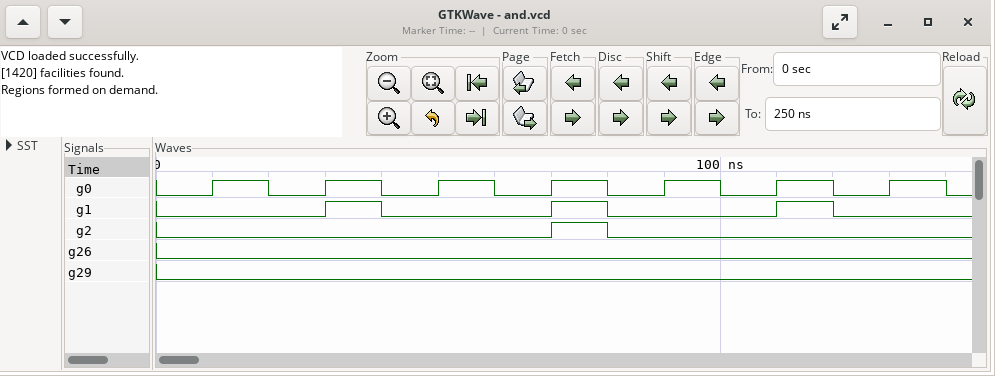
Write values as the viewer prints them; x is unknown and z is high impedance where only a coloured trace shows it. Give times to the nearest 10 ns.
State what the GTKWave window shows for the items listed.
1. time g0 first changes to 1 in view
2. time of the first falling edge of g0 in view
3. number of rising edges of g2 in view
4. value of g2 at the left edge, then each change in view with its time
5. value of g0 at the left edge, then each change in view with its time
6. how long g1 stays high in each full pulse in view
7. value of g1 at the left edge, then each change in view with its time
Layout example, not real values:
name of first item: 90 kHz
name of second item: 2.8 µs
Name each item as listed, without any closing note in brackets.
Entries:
time g0 first changes to 1 in view: 10 ns
time of the first falling edge of g0 in view: 20 ns
number of rising edges of g2 in view: 1
value of g2 at the left edge, then each change in view with its time: 0, 1 at 70 ns, 0 at 80 ns
value of g0 at the left edge, then each change in view with its time: 0, 1 at 10 ns, 0 at 20 ns, 1 at 30 ns, 0 at 40 ns, 1 at 50 ns, 0 at 60 ns, 1 at 70 ns, 0 at 80 ns, 1 at 90 ns, 0 at 100 ns, 1 at 110 ns, 0 at 120 ns, 1 at 130 ns, 0 at 140 ns
how long g1 stays high in each full pulse in view: 10 ns, 10 ns, 10 ns
value of g1 at the left edge, then each change in view with its time: 0, 1 at 30 ns, 0 at 40 ns, 1 at 70 ns, 0 at 80 ns, 1 at 110 ns, 0 at 120 ns
